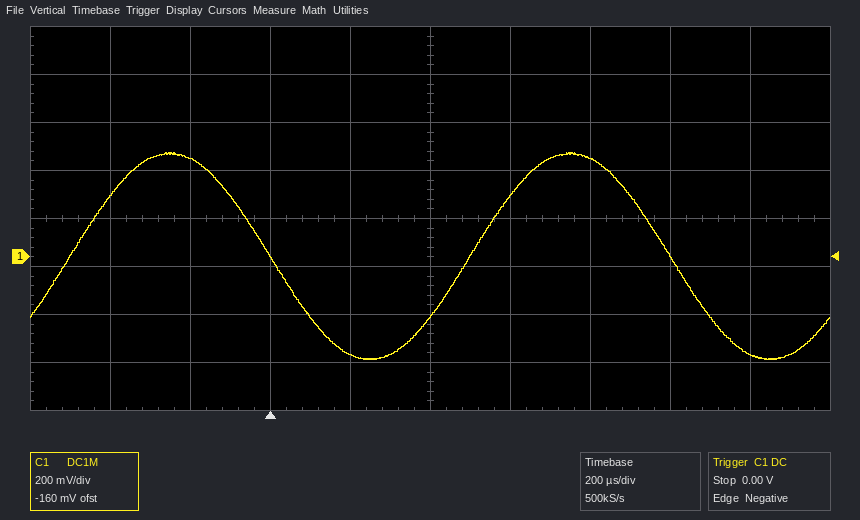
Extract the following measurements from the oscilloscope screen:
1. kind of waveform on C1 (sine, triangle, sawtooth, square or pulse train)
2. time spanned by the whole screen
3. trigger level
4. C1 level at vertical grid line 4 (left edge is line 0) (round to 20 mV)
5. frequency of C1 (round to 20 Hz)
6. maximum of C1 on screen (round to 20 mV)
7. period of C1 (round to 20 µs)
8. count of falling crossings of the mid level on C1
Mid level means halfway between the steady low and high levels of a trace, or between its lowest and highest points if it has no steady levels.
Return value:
sine
2 ms
0.00 V
-400 mV
1.00 kHz
440 mV
1.00 ms
2
